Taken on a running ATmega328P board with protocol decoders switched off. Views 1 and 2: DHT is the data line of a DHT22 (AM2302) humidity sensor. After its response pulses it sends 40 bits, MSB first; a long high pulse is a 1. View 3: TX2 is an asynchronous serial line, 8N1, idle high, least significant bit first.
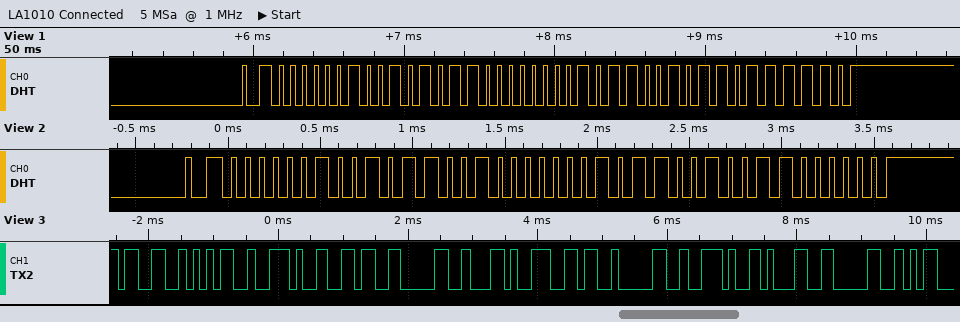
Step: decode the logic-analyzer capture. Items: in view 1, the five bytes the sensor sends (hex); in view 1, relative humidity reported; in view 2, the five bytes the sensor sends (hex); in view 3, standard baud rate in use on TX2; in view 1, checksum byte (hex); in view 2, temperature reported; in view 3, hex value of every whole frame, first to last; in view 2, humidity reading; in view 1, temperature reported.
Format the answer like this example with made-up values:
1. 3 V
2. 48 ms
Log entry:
1. 02 56 01 65 BE
2. 59.8 %
3. 02 59 01 64 C0
4. 9600 baud
5. 0xBE
6. 35.6 °C
7. 0x33 0x35 0x2E 0x36 0x30 0x2C 0x36 0x30 0x2E 0x31 0x30
8. 60.1 %
9. 35.7 °C
